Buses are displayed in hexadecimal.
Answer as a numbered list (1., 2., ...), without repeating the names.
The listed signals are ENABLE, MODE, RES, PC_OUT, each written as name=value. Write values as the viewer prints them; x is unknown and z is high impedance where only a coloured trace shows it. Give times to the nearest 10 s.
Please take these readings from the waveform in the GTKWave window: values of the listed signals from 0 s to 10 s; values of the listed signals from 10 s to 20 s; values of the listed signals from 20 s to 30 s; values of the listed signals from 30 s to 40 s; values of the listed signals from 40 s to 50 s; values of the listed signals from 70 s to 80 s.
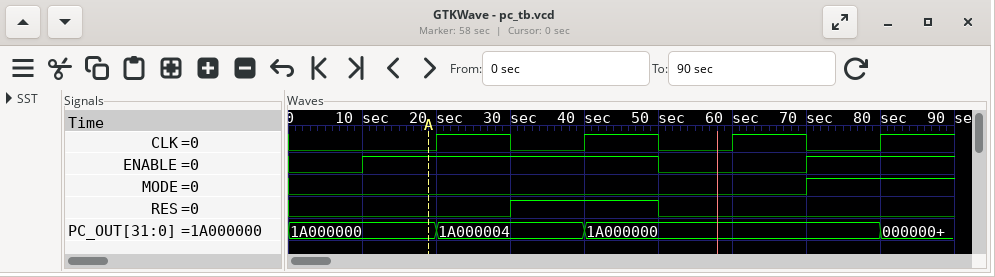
1. ENABLE=0, MODE=0, RES=0, PC_OUT=1A000000
2. ENABLE=1, MODE=0, RES=0, PC_OUT=1A000000
3. ENABLE=1, MODE=0, RES=0, PC_OUT=1A000004
4. ENABLE=1, MODE=0, RES=1, PC_OUT=1A000004
5. ENABLE=1, MODE=0, RES=1, PC_OUT=1A000000
6. ENABLE=1, MODE=1, RES=0, PC_OUT=1A000000
